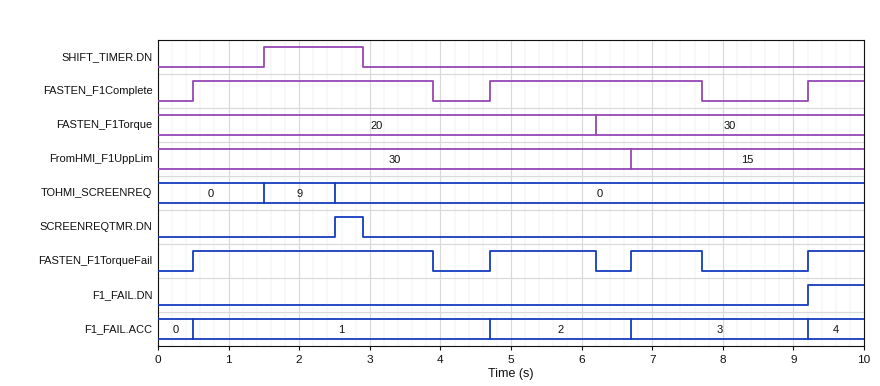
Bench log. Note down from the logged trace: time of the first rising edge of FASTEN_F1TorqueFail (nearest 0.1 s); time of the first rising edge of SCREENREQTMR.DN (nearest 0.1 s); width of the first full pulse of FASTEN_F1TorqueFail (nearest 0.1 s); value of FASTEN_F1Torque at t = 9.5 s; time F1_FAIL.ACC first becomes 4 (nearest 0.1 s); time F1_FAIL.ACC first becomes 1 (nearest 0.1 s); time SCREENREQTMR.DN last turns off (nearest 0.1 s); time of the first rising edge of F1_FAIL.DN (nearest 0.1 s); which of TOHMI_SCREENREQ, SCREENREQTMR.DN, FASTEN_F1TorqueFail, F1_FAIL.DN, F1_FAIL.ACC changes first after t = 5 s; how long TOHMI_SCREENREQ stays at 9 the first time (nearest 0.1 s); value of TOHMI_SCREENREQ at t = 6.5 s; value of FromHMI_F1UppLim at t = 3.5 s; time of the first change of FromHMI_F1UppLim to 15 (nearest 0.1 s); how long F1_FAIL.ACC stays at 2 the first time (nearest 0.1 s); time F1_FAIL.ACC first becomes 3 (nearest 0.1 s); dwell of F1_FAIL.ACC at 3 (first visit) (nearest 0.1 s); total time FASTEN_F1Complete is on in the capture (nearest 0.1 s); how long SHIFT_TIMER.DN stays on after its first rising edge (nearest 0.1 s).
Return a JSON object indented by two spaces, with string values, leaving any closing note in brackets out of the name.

{
  "time of the first rising edge of FASTEN_F1TorqueFail": "0.5 s",
  "time of the first rising edge of SCREENREQTMR.DN": "2.5 s",
  "width of the first full pulse of FASTEN_F1TorqueFail": "3.4 s",
  "value of FASTEN_F1Torque at t = 9.5 s": "30",
  "time F1_FAIL.ACC first becomes 4": "9.2 s",
  "time F1_FAIL.ACC first becomes 1": "0.5 s",
  "time SCREENREQTMR.DN last turns off": "2.9 s",
  "time of the first rising edge of F1_FAIL.DN": "9.2 s",
  "which of TOHMI_SCREENREQ, SCREENREQTMR.DN, FASTEN_F1TorqueFail, F1_FAIL.DN, F1_FAIL.ACC changes first after t = 5 s": "FASTEN_F1TorqueFail",
  "how long TOHMI_SCREENREQ stays at 9 the first time": "1.0 s",
  "value of TOHMI_SCREENREQ at t = 6.5 s": "0",
  "value of FromHMI_F1UppLim at t = 3.5 s": "30",
  "time of the first change of FromHMI_F1UppLim to 15": "6.7 s",
  "how long F1_FAIL.ACC stays at 2 the first time": "2.0 s",
  "time F1_FAIL.ACC first becomes 3": "6.7 s",
  "dwell of F1_FAIL.ACC at 3 (first visit)": "2.5 s",
  "total time FASTEN_F1Complete is on in the capture": "7.2 s",
  "how long SHIFT_TIMER.DN stays on after its first rising edge": "1.4 s"
}
